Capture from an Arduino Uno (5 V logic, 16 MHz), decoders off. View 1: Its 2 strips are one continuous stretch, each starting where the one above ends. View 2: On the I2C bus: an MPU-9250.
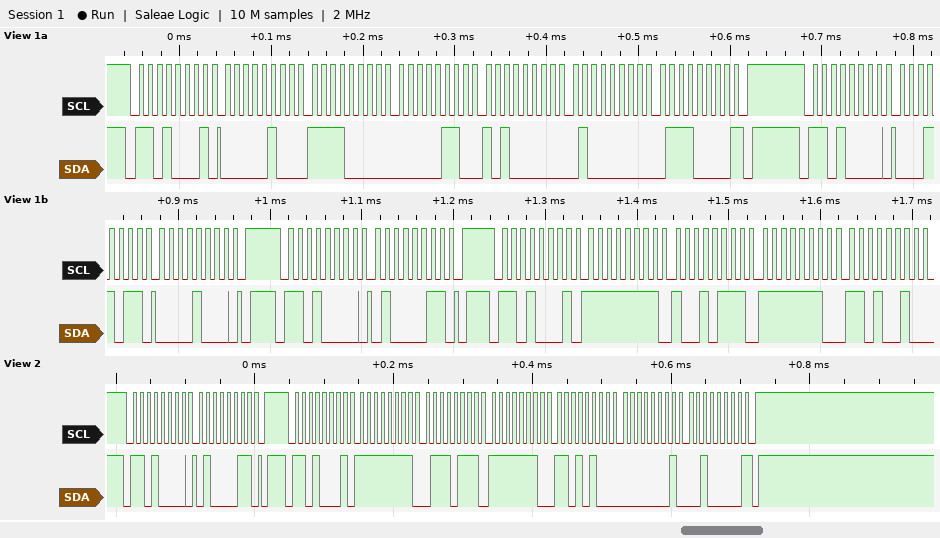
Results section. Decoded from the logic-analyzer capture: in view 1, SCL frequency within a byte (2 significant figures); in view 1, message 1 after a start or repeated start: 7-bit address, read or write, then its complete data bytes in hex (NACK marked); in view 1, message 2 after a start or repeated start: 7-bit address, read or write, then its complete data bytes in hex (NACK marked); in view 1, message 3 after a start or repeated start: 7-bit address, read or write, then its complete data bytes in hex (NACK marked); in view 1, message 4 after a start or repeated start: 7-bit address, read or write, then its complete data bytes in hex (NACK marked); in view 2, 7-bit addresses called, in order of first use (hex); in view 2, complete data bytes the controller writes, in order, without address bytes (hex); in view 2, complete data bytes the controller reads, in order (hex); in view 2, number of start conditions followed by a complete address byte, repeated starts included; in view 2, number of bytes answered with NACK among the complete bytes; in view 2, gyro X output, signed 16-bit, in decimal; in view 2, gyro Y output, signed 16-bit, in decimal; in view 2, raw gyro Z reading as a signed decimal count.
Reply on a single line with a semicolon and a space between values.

100 kHz; 0x68 read: 04 F0 06 A0 40 70 NACK; 0x68 write: 1B 08; 0x68 write: 43; 0x68 read: FF 97 FE D2; 0x68; 43; FF 77 FE D4 01 20; 2; 1; -137; -300; 288
